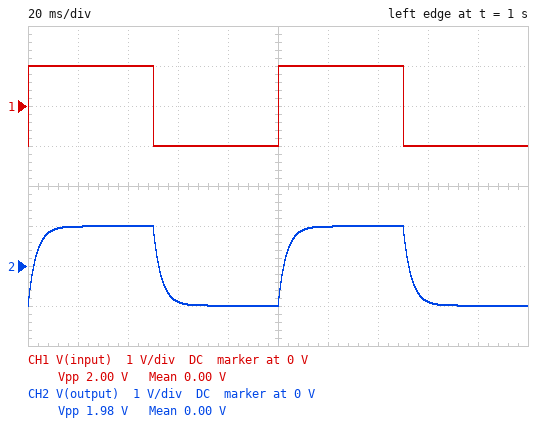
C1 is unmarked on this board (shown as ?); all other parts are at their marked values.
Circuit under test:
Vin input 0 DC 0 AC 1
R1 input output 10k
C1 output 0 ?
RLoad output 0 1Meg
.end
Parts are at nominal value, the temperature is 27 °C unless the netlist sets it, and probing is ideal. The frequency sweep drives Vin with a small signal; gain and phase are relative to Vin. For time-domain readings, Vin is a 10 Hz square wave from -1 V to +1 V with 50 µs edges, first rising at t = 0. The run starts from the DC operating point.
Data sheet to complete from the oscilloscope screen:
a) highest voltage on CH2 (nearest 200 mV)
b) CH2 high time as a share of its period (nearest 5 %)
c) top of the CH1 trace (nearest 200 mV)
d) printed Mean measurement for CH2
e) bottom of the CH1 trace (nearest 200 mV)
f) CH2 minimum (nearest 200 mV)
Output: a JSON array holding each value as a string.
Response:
["1.0 V", "50 %", "1.0 V", "0.00 V", "-1.0 V", "-1.0 V"]
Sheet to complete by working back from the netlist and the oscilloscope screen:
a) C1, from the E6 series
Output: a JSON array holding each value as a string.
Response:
["330 nF"]
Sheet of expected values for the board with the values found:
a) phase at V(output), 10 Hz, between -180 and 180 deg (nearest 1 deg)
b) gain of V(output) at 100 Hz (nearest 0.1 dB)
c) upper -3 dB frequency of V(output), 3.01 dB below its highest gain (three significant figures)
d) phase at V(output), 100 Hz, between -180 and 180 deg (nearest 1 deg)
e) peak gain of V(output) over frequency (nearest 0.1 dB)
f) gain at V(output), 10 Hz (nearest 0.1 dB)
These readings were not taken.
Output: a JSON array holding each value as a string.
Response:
["-12 deg", "-7.3 dB", "48.7 Hz", "-64 deg", "-0.1 dB", "-0.3 dB"]
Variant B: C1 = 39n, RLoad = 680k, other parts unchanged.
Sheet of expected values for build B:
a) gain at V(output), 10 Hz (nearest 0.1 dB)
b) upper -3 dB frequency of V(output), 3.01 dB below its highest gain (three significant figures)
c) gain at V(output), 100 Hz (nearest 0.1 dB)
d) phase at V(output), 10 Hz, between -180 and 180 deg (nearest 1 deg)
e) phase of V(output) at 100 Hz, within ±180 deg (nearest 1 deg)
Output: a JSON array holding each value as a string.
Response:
["-0.1 dB", "414 Hz", "-0.4 dB", "-1 deg", "-14 deg"]
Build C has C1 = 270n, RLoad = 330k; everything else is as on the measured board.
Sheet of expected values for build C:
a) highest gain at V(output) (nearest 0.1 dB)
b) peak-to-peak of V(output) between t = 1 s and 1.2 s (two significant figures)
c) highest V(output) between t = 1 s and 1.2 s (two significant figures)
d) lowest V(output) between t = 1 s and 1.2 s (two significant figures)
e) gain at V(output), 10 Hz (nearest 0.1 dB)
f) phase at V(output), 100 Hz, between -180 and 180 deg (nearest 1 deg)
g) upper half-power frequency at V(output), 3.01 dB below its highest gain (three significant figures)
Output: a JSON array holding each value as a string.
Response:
["-0.3 dB", "1.9 V", "970 mV", "-970 mV", "-0.4 dB", "-59 deg", "60.7 Hz"]
